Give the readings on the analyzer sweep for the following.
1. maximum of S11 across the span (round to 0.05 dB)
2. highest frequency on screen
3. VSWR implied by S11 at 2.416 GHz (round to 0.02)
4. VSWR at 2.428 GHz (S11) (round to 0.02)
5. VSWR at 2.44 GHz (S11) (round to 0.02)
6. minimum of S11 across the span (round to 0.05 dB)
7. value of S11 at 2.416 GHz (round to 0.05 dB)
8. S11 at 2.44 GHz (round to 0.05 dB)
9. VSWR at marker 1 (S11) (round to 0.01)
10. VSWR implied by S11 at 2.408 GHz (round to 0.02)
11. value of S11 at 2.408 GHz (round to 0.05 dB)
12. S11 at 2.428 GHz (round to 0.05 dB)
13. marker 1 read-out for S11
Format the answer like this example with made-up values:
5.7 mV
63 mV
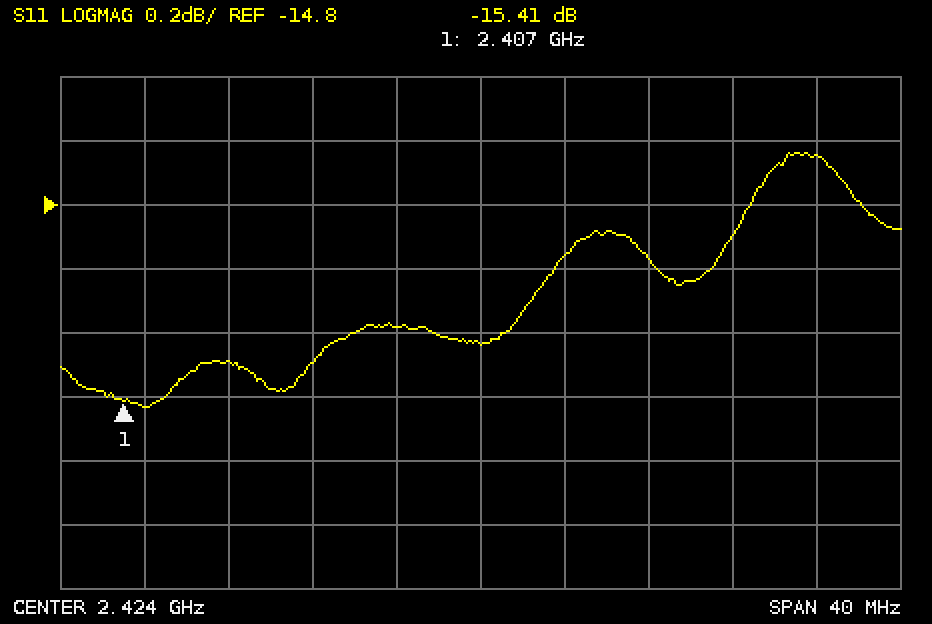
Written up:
-14.65 dB
2.444 GHz
1.42
1.44
1.46
-15.45 dB
-15.30 dB
-14.65 dB
1.41
1.40
-15.45 dB
-14.95 dB
-15.41 dB
